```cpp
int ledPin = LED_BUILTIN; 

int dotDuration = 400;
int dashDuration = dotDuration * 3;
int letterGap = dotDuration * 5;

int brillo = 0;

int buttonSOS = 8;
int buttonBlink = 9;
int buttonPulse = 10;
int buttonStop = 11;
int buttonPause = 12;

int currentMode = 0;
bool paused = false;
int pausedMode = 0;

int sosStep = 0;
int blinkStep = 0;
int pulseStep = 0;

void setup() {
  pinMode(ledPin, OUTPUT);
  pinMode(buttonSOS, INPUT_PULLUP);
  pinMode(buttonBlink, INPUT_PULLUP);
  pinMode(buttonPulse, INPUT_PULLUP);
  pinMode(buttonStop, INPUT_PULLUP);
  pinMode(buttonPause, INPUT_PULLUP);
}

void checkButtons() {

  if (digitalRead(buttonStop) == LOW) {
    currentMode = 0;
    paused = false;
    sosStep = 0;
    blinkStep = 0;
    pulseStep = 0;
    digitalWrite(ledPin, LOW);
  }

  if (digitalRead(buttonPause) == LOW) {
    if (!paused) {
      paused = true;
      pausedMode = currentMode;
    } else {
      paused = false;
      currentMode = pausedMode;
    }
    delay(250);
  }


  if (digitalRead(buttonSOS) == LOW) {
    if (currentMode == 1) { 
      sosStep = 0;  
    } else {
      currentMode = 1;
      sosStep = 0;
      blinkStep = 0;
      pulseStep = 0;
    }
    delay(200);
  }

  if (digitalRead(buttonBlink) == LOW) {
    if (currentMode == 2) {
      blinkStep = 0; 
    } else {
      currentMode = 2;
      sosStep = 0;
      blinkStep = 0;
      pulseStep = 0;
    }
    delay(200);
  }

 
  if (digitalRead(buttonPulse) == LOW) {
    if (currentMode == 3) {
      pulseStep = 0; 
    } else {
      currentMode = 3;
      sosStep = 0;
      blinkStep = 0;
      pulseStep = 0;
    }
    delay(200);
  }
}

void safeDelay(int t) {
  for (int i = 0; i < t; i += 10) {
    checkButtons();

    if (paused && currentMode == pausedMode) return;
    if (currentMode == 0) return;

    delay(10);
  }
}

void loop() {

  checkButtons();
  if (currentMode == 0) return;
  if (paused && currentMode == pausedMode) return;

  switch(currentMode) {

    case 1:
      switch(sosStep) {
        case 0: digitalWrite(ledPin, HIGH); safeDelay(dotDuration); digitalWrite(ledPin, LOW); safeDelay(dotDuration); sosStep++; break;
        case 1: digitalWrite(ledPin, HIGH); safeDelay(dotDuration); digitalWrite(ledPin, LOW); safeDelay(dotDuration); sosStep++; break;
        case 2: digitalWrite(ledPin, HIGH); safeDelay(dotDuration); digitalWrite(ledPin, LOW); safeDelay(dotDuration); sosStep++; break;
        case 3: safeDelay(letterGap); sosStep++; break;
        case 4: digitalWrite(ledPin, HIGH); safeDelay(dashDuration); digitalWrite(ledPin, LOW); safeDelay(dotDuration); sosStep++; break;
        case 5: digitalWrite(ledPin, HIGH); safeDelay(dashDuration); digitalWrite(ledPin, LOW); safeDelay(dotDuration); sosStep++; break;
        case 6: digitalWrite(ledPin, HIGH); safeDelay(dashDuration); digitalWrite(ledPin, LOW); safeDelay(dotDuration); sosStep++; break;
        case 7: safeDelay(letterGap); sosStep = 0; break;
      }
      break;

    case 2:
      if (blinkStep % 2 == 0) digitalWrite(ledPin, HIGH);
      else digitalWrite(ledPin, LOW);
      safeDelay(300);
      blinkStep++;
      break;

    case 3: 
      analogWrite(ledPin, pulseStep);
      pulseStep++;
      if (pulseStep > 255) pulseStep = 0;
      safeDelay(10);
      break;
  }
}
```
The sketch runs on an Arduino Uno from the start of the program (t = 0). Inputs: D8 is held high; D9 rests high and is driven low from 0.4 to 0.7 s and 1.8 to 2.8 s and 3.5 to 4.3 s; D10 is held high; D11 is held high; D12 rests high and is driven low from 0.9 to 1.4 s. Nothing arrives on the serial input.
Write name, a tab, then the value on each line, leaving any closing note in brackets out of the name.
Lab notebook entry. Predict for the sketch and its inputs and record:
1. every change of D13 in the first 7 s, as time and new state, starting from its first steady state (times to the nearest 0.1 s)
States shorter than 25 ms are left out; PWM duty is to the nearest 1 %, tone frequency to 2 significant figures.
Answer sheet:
every change of D13 in the first 7 s, as time and new state, starting from its first steady state	0 s low; 0.6 s high; 1.4 s low; 1.7 s high; 3 s low; 3.3 s high; 4.4 s low; 4.7 s high; 5 s low; 5.3 s high; 5.6 s low; 5.9 s high; 6.2 s low; 6.5 s high; 6.8 s low
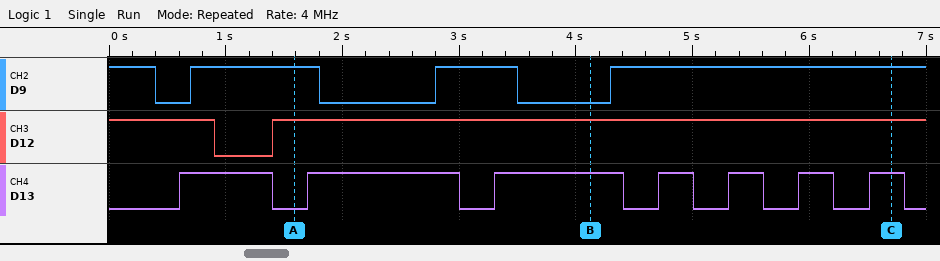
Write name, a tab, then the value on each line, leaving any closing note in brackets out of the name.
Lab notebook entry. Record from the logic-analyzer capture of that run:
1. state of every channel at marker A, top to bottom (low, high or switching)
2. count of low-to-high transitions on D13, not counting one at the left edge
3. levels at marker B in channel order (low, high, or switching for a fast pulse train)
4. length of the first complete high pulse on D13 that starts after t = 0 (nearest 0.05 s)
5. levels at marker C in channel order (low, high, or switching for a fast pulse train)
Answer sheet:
state of every channel at marker A, top to bottom	D9 high, D12 high, D13 low
count of low-to-high transitions on D13, not counting one at the left edge	7
levels at marker B in channel order	D9 low, D12 high, D13 high
length of the first complete high pulse on D13 that starts after t = 0	0.80 s
levels at marker C in channel order	D9 high, D12 high, D13 high
